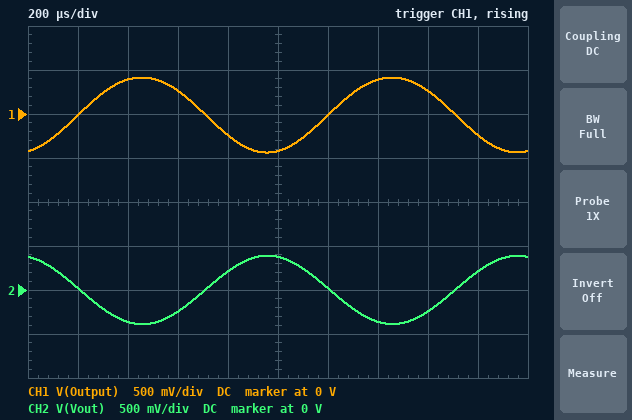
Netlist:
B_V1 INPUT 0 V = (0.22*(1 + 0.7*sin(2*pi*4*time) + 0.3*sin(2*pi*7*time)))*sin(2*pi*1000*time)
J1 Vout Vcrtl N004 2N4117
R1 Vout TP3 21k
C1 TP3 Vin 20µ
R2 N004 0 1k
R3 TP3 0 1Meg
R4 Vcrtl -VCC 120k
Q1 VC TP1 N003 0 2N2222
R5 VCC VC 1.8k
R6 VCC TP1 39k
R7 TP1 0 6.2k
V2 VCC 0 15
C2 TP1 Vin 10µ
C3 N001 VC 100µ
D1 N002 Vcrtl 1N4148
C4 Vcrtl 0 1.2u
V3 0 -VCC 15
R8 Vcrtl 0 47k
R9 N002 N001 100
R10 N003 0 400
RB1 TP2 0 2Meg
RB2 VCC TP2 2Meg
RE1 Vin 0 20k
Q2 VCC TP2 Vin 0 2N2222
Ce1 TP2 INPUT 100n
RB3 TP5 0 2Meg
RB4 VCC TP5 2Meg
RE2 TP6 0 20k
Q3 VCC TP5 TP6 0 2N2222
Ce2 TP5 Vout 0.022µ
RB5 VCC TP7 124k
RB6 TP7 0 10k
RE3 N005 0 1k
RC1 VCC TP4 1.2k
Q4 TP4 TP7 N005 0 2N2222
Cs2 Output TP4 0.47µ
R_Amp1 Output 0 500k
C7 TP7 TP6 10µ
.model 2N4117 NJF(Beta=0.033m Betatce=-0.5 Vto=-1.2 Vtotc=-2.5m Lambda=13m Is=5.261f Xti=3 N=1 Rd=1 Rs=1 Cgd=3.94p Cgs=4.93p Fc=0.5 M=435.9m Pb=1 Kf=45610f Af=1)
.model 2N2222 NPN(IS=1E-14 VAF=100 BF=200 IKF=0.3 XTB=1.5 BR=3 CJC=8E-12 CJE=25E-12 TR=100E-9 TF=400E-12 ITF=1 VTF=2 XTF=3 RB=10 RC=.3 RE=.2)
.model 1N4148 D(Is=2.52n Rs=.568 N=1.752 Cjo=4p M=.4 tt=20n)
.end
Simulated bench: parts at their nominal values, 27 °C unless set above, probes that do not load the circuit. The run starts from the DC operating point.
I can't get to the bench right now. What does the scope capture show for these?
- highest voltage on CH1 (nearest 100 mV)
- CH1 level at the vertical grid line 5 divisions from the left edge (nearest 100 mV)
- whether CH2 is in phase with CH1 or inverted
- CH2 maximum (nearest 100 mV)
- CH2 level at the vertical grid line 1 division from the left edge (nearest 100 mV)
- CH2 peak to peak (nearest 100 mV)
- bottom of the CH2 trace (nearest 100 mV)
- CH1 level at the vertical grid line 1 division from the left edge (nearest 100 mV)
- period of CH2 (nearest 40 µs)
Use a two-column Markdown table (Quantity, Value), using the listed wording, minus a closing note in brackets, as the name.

| Quantity | Value |
|---|---|
| highest voltage on CH1 | 400 mV |
| CH1 level at the vertical grid line 5 divisions from the left edge | -400 mV |
| whether CH2 is in phase with CH1 or inverted | inverted |
| CH2 maximum | 400 mV |
| CH2 level at the vertical grid line 1 division from the left edge | 0 V |
| CH2 peak to peak | 800 mV |
| bottom of the CH2 trace | -400 mV |
| CH1 level at the vertical grid line 1 division from the left edge | 0 V |
| period of CH2 | 1.00 ms |
